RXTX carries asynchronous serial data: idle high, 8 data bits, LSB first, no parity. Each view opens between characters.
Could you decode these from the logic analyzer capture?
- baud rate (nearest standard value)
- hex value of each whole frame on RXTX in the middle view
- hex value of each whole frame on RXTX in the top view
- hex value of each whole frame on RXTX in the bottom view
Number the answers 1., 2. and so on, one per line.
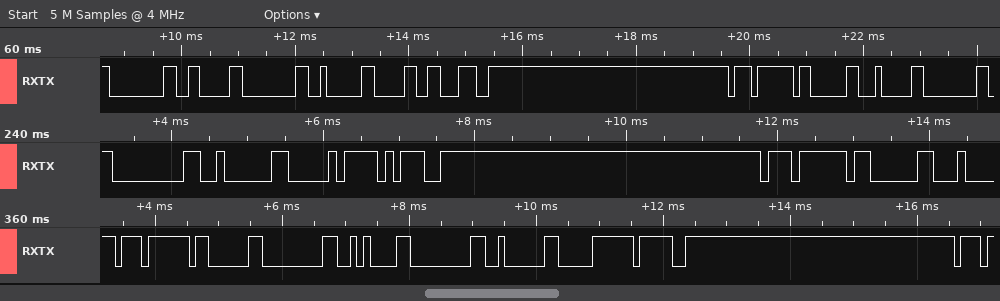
1. 9600 baud
2. 00, 02, D0, 9D, F7, 03
3. 00, 06, 00, 02, 30, 9C, F7, 03, 04, 00
4. F7, 03, 00, 0A, 00, 02, F0, 9F
